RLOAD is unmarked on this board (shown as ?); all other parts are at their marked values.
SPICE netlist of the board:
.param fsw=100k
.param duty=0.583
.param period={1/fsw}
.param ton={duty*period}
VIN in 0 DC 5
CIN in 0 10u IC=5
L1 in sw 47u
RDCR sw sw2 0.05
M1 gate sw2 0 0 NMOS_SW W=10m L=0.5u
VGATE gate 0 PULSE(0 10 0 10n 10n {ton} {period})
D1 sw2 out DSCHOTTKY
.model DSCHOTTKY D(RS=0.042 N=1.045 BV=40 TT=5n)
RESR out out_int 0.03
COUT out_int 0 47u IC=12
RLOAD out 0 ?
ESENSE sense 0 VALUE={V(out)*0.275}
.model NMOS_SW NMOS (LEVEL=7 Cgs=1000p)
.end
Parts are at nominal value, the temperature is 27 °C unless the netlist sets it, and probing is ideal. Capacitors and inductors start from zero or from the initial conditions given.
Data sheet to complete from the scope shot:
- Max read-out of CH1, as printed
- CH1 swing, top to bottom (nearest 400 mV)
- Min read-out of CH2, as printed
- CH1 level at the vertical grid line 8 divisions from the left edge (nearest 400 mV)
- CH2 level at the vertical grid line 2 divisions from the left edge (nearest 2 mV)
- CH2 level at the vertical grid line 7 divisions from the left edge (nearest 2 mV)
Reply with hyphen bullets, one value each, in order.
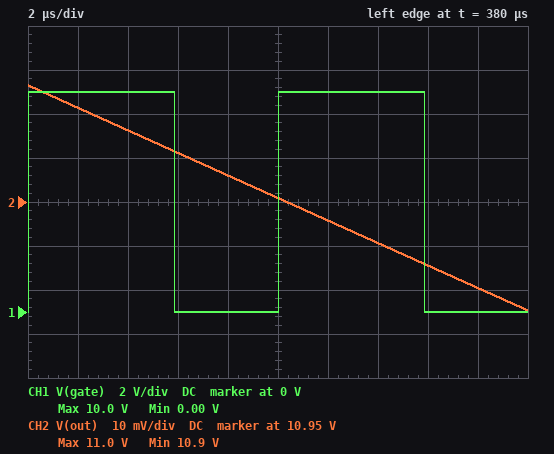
- 10.0 V
- 10.0 V
- 10.9 V
- 0 V
- 10.966 V
- 10.940 V
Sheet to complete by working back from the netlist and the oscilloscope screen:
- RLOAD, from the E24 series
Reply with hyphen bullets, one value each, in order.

- 91 Ω
